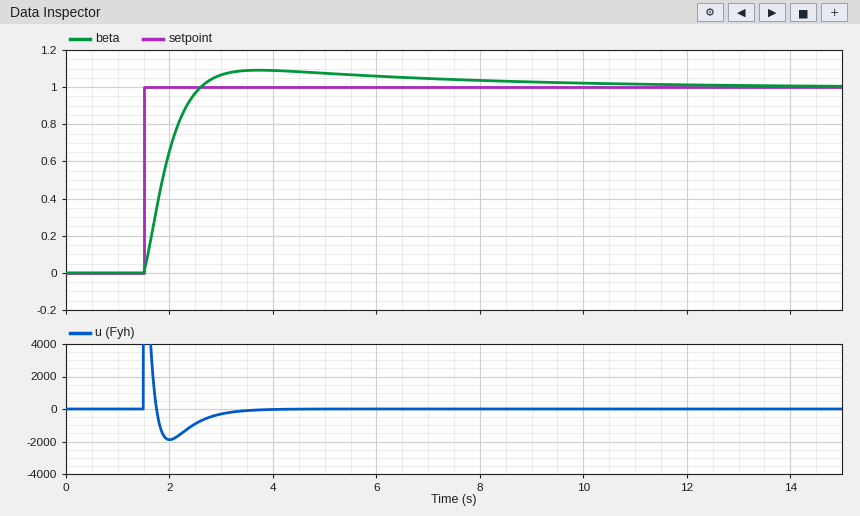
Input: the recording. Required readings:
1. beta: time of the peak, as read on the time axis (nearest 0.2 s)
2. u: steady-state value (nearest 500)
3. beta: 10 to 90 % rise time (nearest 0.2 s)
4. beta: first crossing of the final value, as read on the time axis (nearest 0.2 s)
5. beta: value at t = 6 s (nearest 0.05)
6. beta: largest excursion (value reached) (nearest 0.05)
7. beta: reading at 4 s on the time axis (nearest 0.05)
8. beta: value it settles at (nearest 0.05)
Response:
3.8 s
0
0.8 s
2.6 s
1.05
1.10
1.10
1.00
